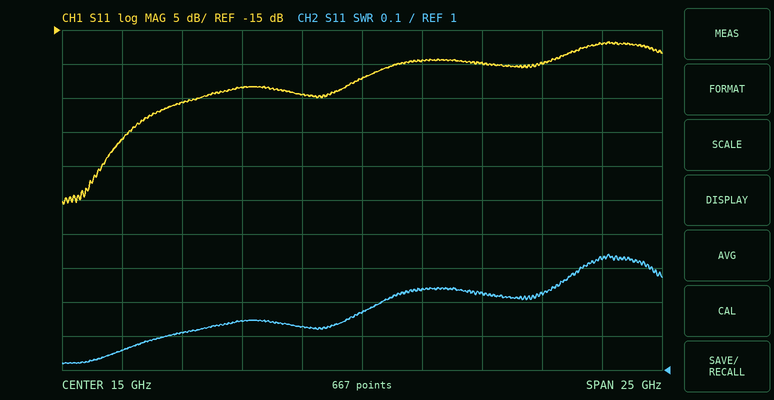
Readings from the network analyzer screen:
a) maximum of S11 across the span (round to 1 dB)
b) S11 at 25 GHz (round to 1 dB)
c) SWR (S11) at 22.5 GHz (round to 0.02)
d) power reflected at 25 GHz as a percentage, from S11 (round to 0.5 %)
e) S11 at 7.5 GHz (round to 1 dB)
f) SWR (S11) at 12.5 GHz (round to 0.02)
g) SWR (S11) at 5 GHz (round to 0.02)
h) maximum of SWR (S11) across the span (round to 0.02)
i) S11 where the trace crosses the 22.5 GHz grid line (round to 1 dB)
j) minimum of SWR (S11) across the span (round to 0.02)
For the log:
-17 dB
-17 dB
1.22
2.0 %
-26 dB
1.12
1.06
1.34
-20 dB
1.02
